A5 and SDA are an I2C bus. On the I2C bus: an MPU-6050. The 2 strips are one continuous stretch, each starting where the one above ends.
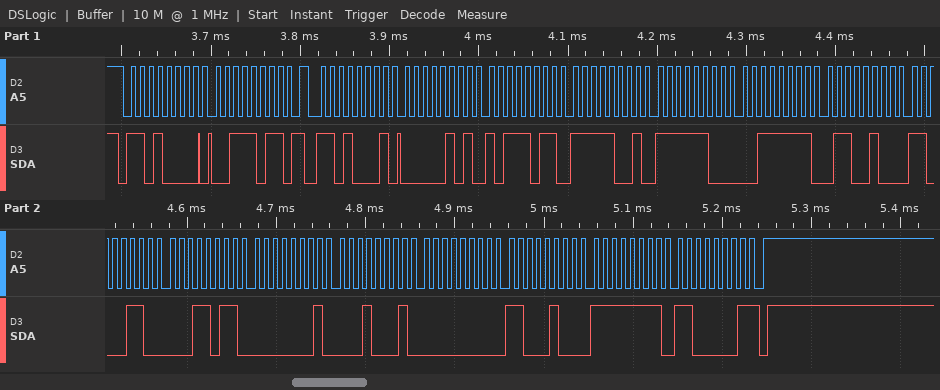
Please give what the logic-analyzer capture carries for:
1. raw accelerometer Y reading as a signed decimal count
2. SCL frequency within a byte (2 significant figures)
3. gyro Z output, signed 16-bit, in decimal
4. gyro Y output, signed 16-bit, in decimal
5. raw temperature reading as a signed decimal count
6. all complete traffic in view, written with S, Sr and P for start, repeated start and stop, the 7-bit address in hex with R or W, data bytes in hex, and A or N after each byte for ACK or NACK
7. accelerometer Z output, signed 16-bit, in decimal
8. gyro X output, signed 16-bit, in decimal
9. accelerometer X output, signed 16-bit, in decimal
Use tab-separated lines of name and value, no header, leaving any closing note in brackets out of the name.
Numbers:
raw accelerometer Y reading as a signed decimal count	-1540
SCL frequency within a byte	100 kHz
gyro Z output, signed 16-bit, in decimal	-63
gyro Y output, signed 16-bit, in decimal	196
raw temperature reading as a signed decimal count	-14821
all complete traffic in view, written with S, Sr and P for start, repeated start and stop, the 7-bit address in hex with R or W, data bytes in hex, and A or N after each byte for ACK or NACK	S 68W A 3B A Sr 68R A 05 A BB A F9 A FC A 3F A 64 A C6 A 1B A 01 A 11 A 00 A C4 A FF A C1 N P
accelerometer Z output, signed 16-bit, in decimal	16228
gyro X output, signed 16-bit, in decimal	273
accelerometer X output, signed 16-bit, in decimal	1467
